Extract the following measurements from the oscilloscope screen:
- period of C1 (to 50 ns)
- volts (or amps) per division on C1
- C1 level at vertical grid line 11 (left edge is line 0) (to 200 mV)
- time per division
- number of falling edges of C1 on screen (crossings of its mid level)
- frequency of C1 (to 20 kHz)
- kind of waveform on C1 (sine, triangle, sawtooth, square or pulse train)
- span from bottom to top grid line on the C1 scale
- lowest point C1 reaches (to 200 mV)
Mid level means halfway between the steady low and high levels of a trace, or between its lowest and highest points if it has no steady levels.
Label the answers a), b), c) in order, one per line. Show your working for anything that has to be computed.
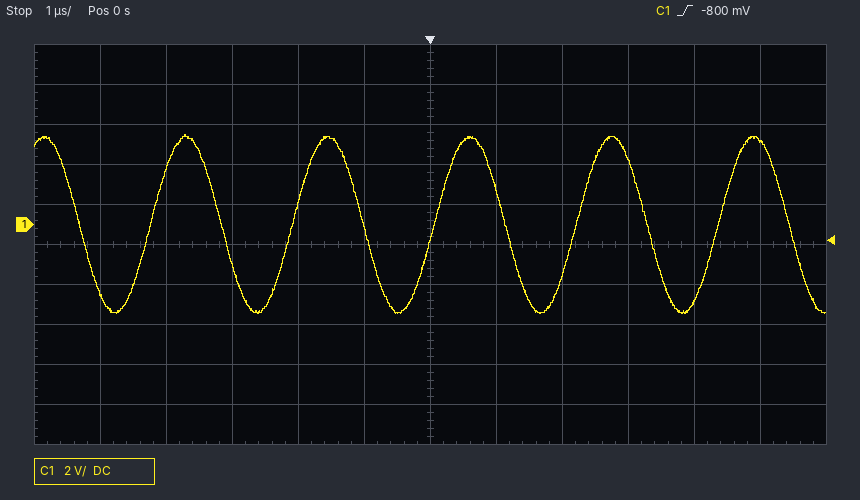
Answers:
a) 2.15 µs
b) 2 V
c) 4.2 V
d) 1 µs
e) 6
f) 1 / 2.15 µs ≈ 465 kHz, so 460 kHz to the nearest 20 kHz
g) sine
h) 20 V
i) -4.4 V
